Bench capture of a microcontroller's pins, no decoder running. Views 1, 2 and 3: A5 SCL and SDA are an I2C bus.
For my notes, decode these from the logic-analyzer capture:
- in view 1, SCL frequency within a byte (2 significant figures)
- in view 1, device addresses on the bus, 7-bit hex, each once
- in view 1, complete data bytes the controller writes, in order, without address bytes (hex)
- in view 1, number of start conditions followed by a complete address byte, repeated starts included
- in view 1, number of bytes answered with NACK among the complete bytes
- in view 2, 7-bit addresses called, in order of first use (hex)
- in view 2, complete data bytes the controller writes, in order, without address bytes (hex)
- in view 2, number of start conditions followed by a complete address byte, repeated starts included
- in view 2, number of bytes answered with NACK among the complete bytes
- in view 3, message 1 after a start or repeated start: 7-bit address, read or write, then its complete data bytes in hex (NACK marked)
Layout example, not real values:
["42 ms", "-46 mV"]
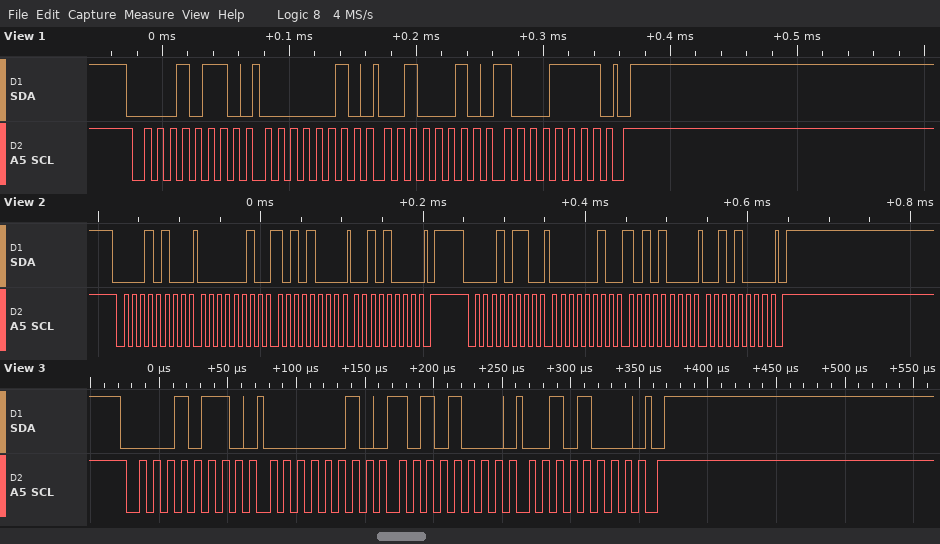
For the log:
["100 kHz", "0x0B", "02 22 8F", "1", "0", "0x0A 0x0B", "02 A8 28 02 A8 28", "2", "0", "0x0B write: 02 A8 28"]
